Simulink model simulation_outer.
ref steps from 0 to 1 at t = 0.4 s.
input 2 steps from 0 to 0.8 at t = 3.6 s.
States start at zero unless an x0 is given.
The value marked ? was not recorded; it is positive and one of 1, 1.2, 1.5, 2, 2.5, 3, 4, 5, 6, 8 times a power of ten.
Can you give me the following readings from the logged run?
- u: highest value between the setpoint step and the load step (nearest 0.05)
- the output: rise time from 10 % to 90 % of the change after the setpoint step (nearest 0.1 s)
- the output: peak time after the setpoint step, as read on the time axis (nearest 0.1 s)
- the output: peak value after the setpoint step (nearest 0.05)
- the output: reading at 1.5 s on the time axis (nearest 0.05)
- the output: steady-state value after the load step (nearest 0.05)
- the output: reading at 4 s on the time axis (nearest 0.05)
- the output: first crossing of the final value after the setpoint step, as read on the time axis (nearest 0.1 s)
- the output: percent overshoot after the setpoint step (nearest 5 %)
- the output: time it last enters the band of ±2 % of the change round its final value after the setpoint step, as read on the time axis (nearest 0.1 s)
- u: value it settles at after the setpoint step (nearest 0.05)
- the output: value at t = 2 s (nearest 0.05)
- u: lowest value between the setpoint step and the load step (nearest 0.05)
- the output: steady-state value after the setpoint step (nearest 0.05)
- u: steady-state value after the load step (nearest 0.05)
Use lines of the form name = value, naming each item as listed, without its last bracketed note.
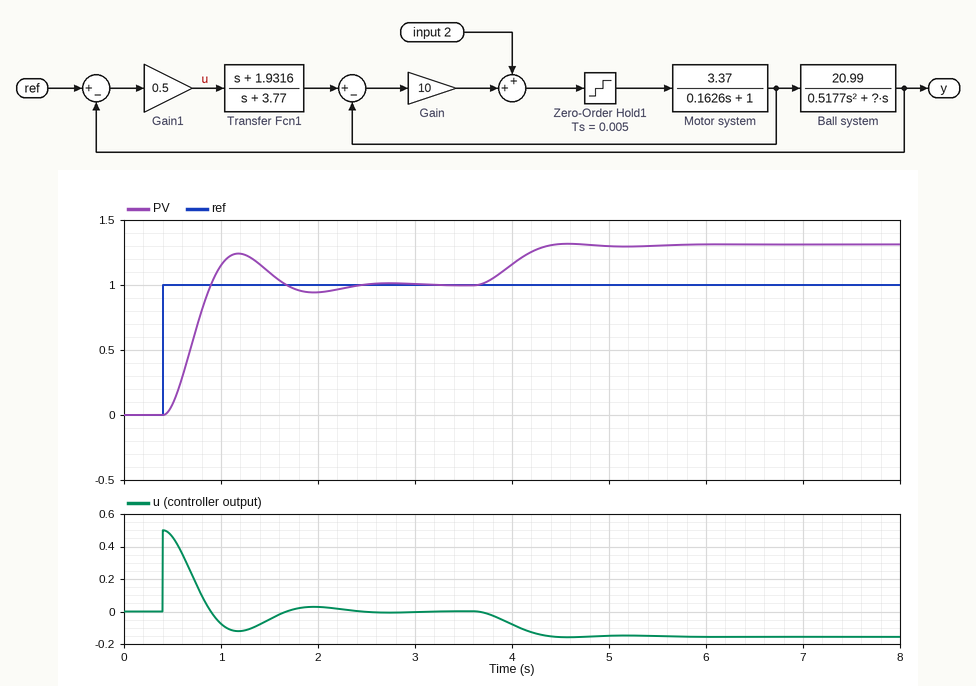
u: highest value between the setpoint step and the load step = 0.50
the output: rise time from 10 % to 90 % of the change after the setpoint step = 0.3 s
the output: peak time after the setpoint step, as read on the time axis = 1.2 s
the output: peak value after the setpoint step = 1.25
the output: reading at 1.5 s on the time axis = 1.10
the output: steady-state value after the load step = 1.30
the output: reading at 4 s on the time axis = 1.15
the output: first crossing of the final value after the setpoint step, as read on the time axis = 0.9 s
the output: percent overshoot after the setpoint step = 25 %
the output: time it last enters the band of ±2 % of the change round its final value after the setpoint step, as read on the time axis = 2.3 s
u: value it settles at after the setpoint step = 0.00
the output: value at t = 2 s = 0.95
u: lowest value between the setpoint step and the load step = -0.10
the output: steady-state value after the setpoint step = 1.00
u: steady-state value after the load step = -0.15
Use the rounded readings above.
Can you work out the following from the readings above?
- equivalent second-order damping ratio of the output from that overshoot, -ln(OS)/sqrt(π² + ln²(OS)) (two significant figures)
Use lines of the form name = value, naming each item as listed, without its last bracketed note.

equivalent second-order damping ratio of the output from that overshoot, -ln(OS)/sqrt(π² + ln²(OS)) = 0.40
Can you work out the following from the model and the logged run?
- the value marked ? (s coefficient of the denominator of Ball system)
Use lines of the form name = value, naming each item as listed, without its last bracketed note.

the value marked ? = 1
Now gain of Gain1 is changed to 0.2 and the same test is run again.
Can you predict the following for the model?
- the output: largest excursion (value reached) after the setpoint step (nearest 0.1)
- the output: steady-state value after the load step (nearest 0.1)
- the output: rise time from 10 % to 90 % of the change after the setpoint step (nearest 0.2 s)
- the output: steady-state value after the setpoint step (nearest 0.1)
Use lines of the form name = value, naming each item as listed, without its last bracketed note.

the output: largest excursion (value reached) after the setpoint step = 1.1
the output: steady-state value after the load step = 1.8
the output: rise time from 10 % to 90 % of the change after the setpoint step = 0.8 s
the output: steady-state value after the setpoint step = 1.0
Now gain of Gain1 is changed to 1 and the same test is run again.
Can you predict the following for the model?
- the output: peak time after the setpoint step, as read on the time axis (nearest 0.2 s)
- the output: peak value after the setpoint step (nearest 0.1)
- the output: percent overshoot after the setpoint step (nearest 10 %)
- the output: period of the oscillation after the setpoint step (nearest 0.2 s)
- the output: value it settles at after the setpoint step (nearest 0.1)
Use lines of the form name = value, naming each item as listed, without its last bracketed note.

the output: peak time after the setpoint step, as read on the time axis = 1.0 s
the output: peak value after the setpoint step = 1.4
the output: percent overshoot after the setpoint step = 40 %
the output: period of the oscillation after the setpoint step = 1.0 s
the output: value it settles at after the setpoint step = 1.0
